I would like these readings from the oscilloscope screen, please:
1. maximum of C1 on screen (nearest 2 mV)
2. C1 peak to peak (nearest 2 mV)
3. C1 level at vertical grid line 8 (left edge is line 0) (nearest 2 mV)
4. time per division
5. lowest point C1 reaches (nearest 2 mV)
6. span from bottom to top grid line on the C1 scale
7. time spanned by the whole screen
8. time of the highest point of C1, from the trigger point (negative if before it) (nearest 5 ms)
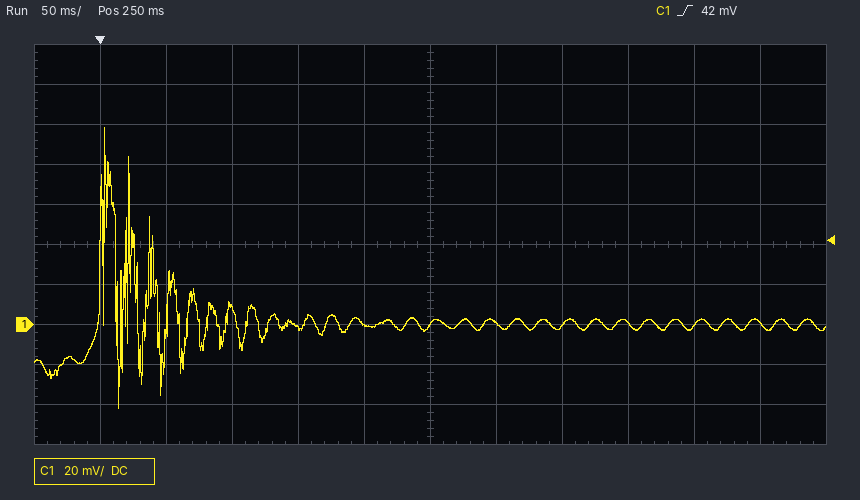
98 mV
140 mV
0 mV
50 ms
-42 mV
200 mV
600 ms
+5 ms
